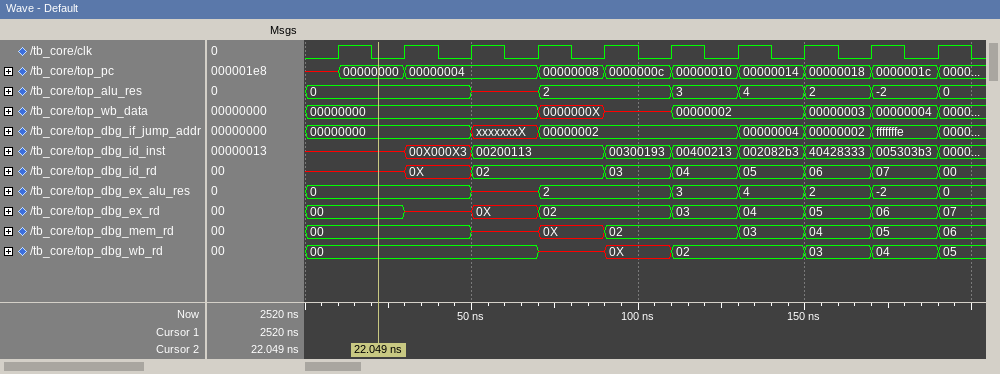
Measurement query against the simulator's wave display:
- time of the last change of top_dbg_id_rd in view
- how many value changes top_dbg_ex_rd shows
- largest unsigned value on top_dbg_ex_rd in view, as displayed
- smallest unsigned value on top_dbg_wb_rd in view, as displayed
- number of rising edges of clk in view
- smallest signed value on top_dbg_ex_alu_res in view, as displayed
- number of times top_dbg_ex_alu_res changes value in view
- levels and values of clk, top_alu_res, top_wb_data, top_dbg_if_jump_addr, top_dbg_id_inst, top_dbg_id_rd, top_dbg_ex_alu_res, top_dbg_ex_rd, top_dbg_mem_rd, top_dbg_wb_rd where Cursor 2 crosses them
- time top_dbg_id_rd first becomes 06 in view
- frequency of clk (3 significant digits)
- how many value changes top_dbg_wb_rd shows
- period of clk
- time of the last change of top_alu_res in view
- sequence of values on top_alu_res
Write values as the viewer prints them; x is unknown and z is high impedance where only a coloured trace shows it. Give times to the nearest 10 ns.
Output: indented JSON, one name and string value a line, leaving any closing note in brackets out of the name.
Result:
{
  "time of the last change of top_dbg_id_rd in view": "190 ns",
  "how many value changes top_dbg_ex_rd shows": "8",
  "largest unsigned value on top_dbg_ex_rd in view, as displayed": "07",
  "smallest unsigned value on top_dbg_wb_rd in view, as displayed": "00",
  "number of rising edges of clk in view": "10",
  "smallest signed value on top_dbg_ex_alu_res in view, as displayed": "-2",
  "number of times top_dbg_ex_alu_res changes value in view": "7",
  "levels and values of clk, top_alu_res, top_wb_data, top_dbg_if_jump_addr, top_dbg_id_inst, top_dbg_id_rd, top_dbg_ex_alu_res, top_dbg_ex_rd, top_dbg_mem_rd, top_dbg_wb_rd where Cursor 2 crosses them": "clk=0, top_alu_res=0, top_wb_data=00000000, top_dbg_if_jump_addr=00000000, top_dbg_id_inst=x, top_dbg_id_rd=x, top_dbg_ex_alu_res=0, top_dbg_ex_rd=00, top_dbg_mem_rd=00, top_dbg_wb_rd=00",
  "time top_dbg_id_rd first becomes 06 in view": "150 ns",
  "frequency of clk": "50.0 MHz",
  "how many value changes top_dbg_wb_rd shows": "6",
  "period of clk": "20 ns",
  "time of the last change of top_alu_res in view": "190 ns",
  "sequence of values on top_alu_res": "0, x, 2, 3, 4, 2, -2, 0"
}
